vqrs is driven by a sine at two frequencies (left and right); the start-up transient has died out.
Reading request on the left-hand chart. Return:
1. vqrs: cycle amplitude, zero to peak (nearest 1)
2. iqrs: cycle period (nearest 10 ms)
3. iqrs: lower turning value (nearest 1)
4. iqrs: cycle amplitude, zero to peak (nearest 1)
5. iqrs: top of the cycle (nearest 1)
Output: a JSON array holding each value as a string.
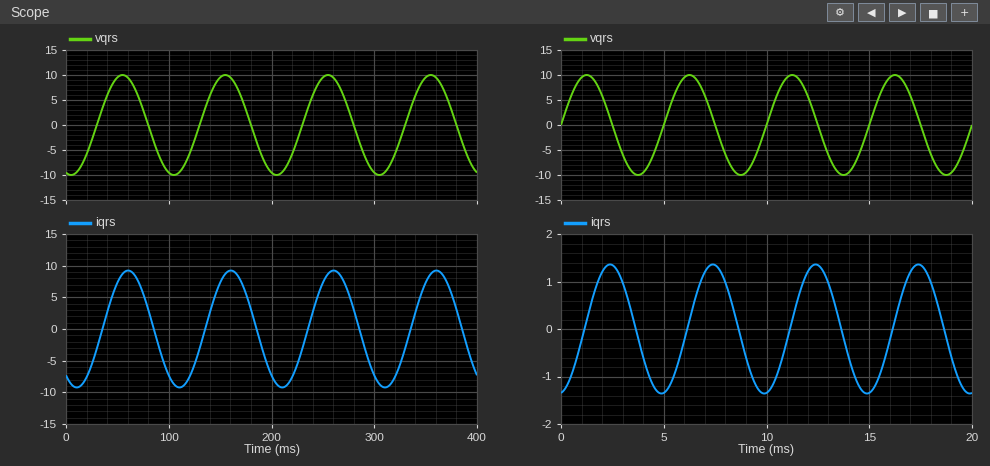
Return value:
["10", "100 ms", "-9", "9", "9"]
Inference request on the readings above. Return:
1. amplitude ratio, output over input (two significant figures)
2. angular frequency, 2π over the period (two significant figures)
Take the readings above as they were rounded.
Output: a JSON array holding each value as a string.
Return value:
["0.90", "0.063 rad/ms"]
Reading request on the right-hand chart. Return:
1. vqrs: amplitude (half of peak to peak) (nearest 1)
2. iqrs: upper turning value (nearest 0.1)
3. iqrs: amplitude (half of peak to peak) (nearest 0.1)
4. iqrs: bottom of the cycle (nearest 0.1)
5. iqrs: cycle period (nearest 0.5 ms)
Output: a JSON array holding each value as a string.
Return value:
["10", "1.4", "1.4", "-1.4", "5.0 ms"]
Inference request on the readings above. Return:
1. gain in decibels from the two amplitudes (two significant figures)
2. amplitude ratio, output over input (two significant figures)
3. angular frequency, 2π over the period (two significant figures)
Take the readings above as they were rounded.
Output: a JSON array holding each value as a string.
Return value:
["-17 dB", "0.14", "1.3 rad/ms"]
